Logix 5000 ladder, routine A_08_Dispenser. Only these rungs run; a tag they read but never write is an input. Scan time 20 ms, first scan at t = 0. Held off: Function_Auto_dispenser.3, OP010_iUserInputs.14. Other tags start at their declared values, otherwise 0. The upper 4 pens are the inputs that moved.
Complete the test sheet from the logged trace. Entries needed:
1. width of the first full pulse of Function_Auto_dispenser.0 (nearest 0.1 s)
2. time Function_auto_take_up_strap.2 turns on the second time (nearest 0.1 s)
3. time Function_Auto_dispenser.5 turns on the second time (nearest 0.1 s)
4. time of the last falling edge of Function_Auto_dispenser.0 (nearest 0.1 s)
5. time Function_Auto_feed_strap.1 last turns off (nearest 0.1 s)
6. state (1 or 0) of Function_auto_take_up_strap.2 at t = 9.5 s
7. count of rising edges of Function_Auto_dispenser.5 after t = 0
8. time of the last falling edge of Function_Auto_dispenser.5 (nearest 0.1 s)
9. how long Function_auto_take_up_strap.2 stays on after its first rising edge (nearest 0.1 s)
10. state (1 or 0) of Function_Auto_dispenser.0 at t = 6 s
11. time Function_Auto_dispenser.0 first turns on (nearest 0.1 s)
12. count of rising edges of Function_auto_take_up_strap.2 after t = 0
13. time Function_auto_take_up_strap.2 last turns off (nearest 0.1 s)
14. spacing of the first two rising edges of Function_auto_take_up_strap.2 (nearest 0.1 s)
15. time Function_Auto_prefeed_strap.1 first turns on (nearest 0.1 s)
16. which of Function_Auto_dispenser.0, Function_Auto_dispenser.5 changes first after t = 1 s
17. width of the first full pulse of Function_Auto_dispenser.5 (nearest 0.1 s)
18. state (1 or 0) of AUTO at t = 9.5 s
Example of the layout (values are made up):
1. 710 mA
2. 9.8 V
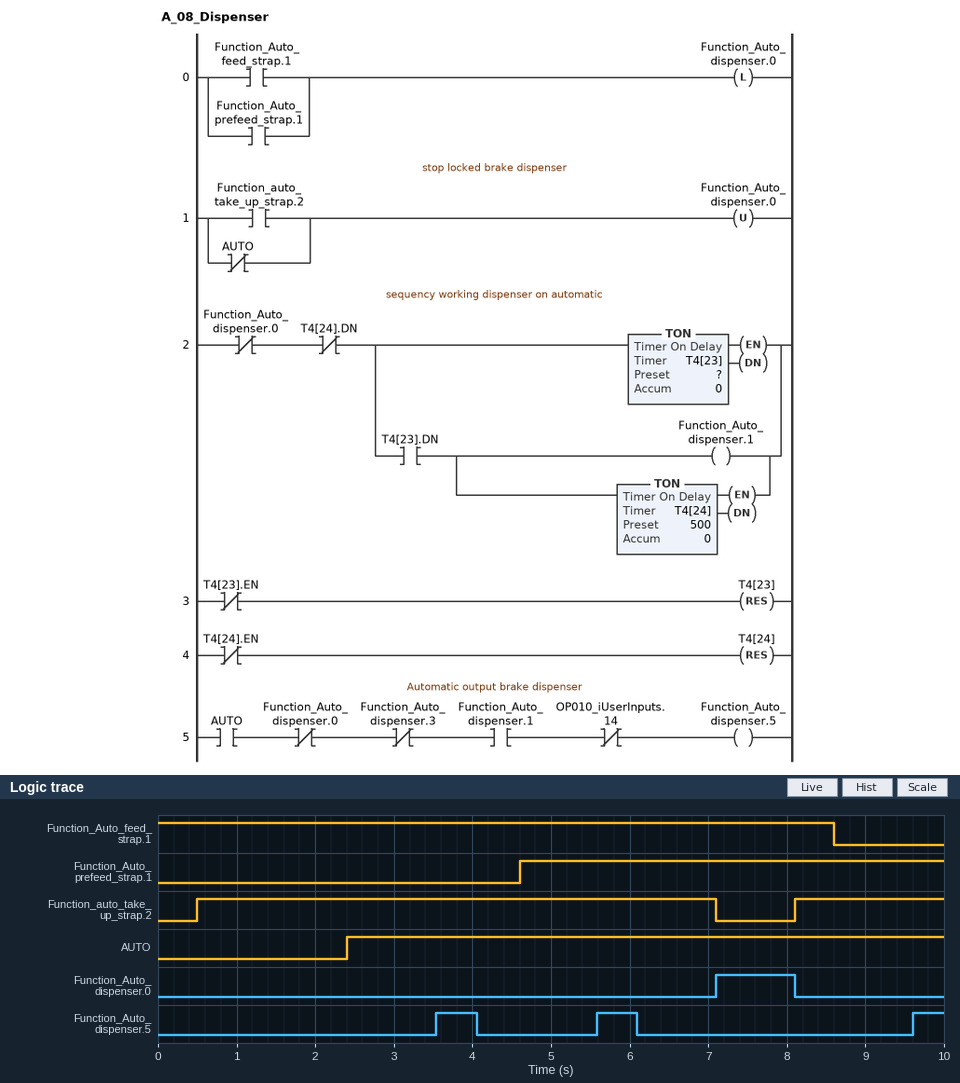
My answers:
1. 1.0 s
2. 8.1 s
3. 5.6 s
4. 8.1 s
5. 8.6 s
6. 1
7. 3
8. 6.1 s
9. 6.6 s
10. 0
11. 7.1 s
12. 2
13. 7.1 s
14. 7.6 s
15. 4.6 s
16. Function_Auto_dispenser.5
17. 0.5 s
18. 1
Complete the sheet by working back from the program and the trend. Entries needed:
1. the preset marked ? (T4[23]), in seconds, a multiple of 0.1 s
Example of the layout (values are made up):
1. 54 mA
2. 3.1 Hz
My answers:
1. 1.5 s
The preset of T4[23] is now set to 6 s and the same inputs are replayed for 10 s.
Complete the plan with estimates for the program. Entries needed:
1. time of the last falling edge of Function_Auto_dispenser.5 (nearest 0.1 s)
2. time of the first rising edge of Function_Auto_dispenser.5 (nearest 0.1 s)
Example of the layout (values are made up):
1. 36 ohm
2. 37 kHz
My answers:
1. 6.5 s
2. 6.0 s
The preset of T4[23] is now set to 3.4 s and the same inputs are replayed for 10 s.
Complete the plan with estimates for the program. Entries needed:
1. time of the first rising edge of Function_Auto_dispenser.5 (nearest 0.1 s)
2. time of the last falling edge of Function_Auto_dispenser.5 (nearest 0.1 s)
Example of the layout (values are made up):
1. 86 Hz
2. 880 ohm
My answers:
1. 3.4 s
2. 3.9 s
